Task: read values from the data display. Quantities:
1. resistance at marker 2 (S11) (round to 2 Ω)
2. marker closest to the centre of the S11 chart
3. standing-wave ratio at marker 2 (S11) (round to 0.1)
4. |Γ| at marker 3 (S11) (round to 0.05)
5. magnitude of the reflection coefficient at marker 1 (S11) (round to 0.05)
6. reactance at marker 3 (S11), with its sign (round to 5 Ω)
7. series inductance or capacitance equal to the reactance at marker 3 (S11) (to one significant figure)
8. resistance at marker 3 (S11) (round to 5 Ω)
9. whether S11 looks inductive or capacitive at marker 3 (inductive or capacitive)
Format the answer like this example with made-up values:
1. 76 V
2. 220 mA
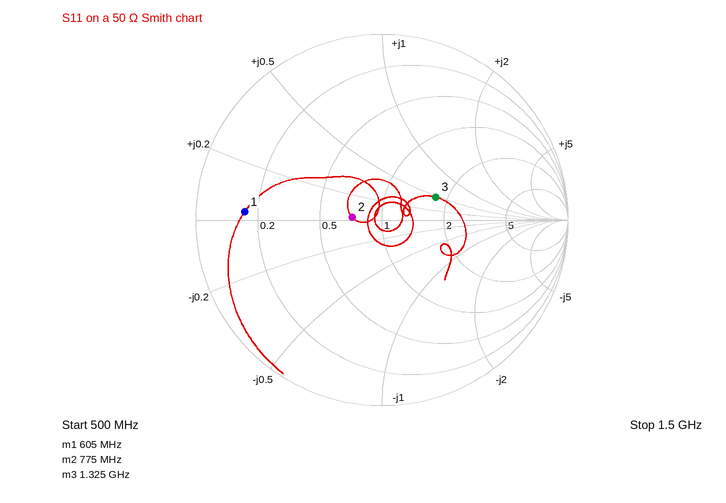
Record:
1. 36 Ω
2. marker 2
3. 1.4
4. 0.30
5. 0.75
6. +25 Ω
7. 3 nH
8. 85 Ω
9. inductive
